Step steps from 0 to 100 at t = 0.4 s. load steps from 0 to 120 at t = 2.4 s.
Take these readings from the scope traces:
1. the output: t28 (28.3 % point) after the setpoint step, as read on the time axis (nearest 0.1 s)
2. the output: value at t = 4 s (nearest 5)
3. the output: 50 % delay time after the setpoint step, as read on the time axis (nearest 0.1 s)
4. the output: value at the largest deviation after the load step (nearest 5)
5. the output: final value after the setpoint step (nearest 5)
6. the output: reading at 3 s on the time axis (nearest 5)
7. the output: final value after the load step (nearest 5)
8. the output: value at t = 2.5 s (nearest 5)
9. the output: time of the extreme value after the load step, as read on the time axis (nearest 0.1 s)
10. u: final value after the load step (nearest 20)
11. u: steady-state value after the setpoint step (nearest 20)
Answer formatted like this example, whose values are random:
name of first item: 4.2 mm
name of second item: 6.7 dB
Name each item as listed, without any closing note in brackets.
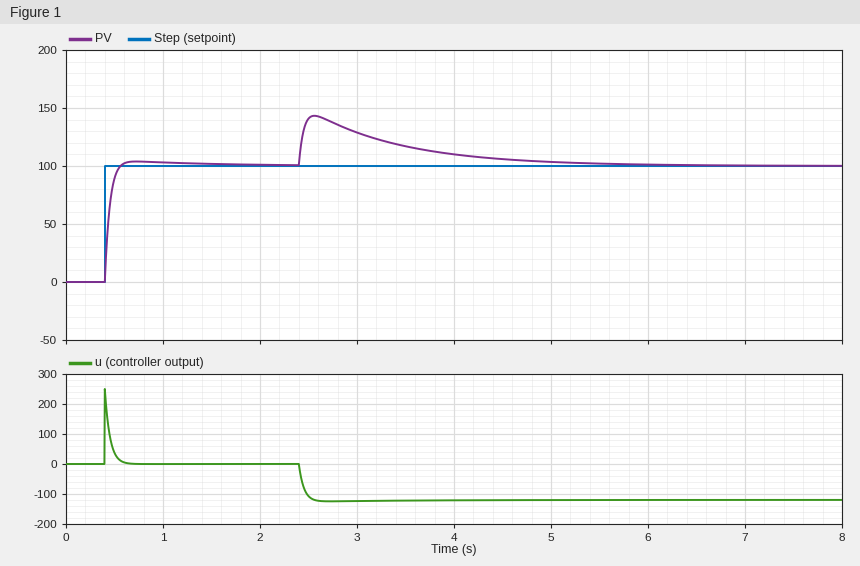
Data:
the output: t28 (28.3 % point) after the setpoint step, as read on the time axis: 0.4 s
the output: value at t = 4 s: 110
the output: 50 % delay time after the setpoint step, as read on the time axis: 0.4 s
the output: value at the largest deviation after the load step: 145
the output: final value after the setpoint step: 100
the output: reading at 3 s on the time axis: 130
the output: final value after the load step: 100
the output: value at t = 2.5 s: 140
the output: time of the extreme value after the load step, as read on the time axis: 2.6 s
u: final value after the load step: -120
u: steady-state value after the setpoint step: 0
